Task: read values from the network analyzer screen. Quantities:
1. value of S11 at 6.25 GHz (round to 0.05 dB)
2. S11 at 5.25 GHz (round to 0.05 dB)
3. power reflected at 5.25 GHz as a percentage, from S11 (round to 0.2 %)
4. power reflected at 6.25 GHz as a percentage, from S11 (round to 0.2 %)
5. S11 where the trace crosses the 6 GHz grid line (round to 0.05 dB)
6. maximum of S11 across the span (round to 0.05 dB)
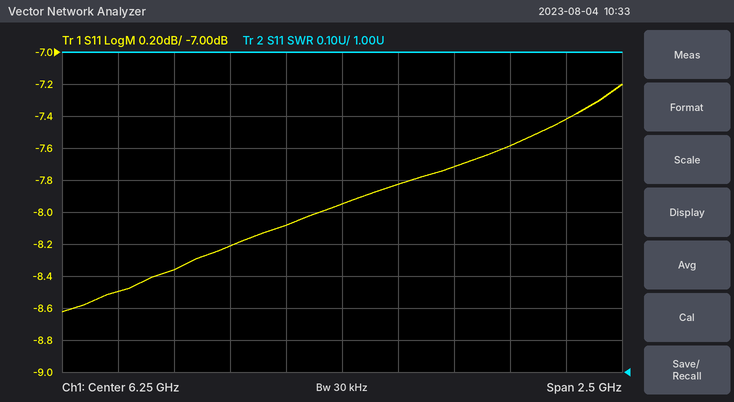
-7.95 dB
-8.50 dB
14.2 %
16.0 %
-8.10 dB
-7.20 dB
